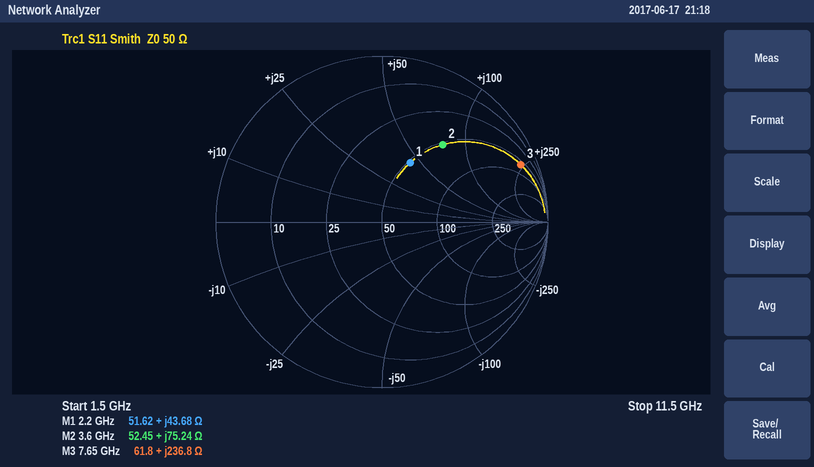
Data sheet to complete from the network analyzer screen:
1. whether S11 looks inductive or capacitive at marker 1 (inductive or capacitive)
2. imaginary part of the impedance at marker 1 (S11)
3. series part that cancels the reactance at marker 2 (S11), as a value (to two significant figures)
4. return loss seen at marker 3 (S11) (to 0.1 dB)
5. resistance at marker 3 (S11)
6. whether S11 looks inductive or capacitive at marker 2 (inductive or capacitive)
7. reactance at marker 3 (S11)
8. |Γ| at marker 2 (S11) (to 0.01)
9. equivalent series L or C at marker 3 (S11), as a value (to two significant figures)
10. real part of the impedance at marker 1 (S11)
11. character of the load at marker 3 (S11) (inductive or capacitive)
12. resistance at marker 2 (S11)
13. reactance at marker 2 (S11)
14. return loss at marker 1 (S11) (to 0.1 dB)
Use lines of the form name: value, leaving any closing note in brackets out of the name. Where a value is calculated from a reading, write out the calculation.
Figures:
whether S11 looks inductive or capacitive at marker 1: inductive
imaginary part of the impedance at marker 1: +43.68 Ω
series part that cancels the reactance at marker 2 (S11), as a value: C = 1/(2π × 3.6 GHz × 75.24 Ω) ≈ 588 fF, so 590 fF to two significant figures
return loss seen at marker 3 (S11): 0.9 dB
resistance at marker 3: 61.8 Ω
whether S11 looks inductive or capacitive at marker 2: inductive
reactance at marker 3: +236.8 Ω
|Γ| at marker 2 (S11): 0.59
equivalent series L or C at marker 3 (S11), as a value: L = 236.8 Ω/(2π × 7.65 GHz) ≈ 4.9 nH
real part of the impedance at marker 1: 51.62 Ω
character of the load at marker 3 (S11): inductive
resistance at marker 2: 52.45 Ω
reactance at marker 2: +75.24 Ω
return loss at marker 1 (S11): 8.1 dB
